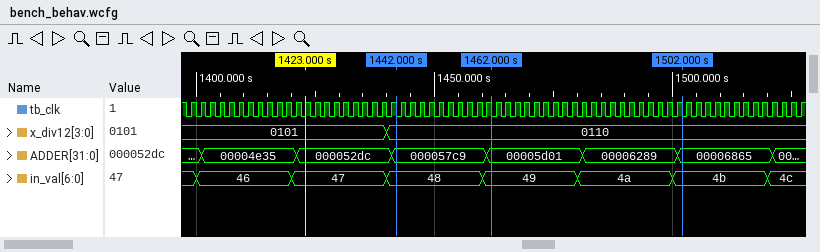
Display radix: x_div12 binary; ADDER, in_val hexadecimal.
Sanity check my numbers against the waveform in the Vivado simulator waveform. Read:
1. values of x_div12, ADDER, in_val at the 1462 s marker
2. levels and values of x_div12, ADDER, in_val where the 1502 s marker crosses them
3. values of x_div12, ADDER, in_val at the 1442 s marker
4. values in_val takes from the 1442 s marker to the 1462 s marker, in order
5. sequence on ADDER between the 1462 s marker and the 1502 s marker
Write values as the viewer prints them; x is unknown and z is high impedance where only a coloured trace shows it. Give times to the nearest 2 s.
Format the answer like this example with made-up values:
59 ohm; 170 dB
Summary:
x_div12=0110, ADDER=00005d01, in_val=49; x_div12=0110, ADDER=00006865, in_val=4b; x_div12=0110, ADDER=000057c9, in_val=48; 48, 49; 00005d01, 00006289, 00006865
